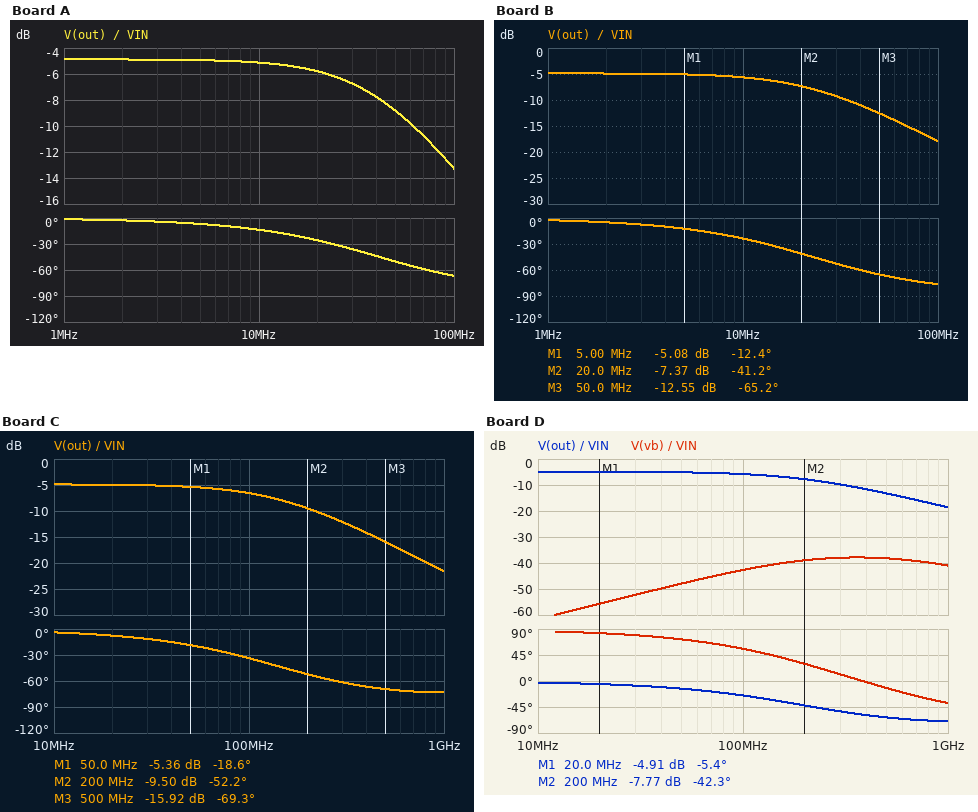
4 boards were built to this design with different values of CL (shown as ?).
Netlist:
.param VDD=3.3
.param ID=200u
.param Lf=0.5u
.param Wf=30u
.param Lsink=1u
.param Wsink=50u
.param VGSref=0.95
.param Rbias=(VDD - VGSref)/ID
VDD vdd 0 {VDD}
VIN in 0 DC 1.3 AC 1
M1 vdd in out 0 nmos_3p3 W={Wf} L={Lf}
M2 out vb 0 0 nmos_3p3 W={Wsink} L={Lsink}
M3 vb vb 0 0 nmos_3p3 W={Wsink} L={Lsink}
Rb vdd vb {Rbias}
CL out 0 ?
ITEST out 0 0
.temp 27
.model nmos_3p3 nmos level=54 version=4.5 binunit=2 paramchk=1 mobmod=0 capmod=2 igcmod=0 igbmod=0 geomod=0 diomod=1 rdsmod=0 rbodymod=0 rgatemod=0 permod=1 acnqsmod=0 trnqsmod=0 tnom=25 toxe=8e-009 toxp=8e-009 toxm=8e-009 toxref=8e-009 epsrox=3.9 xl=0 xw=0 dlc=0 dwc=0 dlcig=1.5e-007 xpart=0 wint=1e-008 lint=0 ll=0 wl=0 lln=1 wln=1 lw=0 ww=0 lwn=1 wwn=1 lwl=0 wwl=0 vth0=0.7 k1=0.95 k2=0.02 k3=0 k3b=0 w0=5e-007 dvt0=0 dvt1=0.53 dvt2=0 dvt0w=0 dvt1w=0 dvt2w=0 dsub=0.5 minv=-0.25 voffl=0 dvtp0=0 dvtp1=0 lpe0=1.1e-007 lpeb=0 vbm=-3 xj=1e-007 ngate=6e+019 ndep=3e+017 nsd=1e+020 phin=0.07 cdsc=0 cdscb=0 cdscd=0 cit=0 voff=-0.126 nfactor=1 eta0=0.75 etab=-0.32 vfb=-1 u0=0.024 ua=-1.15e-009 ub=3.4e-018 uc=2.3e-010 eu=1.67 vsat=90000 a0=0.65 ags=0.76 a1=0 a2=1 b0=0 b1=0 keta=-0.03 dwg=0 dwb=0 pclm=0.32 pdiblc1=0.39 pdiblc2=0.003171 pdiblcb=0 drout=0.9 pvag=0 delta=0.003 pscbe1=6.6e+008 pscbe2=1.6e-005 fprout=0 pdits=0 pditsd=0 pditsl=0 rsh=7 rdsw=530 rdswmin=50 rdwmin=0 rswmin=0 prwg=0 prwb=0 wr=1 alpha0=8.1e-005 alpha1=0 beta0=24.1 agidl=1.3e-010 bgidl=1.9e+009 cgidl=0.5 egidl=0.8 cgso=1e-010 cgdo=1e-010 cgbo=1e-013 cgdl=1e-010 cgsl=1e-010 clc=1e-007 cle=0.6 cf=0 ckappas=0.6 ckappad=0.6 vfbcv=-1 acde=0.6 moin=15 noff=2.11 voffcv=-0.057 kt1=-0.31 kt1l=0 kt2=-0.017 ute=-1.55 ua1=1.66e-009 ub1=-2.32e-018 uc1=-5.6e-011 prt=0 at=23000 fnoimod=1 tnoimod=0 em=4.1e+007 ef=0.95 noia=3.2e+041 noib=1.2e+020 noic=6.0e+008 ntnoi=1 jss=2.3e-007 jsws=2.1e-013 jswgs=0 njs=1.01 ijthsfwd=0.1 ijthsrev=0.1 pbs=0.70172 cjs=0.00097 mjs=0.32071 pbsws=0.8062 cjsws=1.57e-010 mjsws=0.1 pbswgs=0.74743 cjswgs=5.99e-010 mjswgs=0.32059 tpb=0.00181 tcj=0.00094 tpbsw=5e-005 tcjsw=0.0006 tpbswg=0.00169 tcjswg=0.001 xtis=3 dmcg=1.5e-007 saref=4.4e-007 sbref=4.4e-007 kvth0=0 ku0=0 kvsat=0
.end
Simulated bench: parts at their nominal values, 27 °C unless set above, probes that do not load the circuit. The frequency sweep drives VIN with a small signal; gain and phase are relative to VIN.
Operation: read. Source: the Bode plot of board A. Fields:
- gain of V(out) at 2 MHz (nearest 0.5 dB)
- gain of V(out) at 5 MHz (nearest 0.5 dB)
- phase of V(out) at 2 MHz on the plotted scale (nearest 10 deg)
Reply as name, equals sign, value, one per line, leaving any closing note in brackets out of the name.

gain of V(out) at 2 MHz = -5.0 dB
gain of V(out) at 5 MHz = -5.0 dB
phase of V(out) at 2 MHz on the plotted scale = 0 deg
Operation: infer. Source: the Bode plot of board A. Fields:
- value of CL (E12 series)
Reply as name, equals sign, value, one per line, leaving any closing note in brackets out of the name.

value of CL = 8.2 pF
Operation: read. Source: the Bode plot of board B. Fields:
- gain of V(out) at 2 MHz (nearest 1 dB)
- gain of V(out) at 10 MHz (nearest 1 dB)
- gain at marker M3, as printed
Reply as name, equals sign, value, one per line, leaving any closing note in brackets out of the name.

gain of V(out) at 2 MHz = -5 dB
gain of V(out) at 10 MHz = -6 dB
gain at marker M3, as printed = -12.55 dB
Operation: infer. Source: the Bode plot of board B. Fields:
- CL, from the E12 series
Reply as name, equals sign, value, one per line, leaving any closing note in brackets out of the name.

CL, from the E12 series = 15 pF
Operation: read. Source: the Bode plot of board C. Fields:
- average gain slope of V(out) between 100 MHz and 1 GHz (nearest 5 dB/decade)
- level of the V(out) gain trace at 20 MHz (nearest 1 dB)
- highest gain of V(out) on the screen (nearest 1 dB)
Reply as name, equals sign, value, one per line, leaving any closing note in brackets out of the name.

average gain slope of V(out) between 100 MHz and 1 GHz = -15 dB/decade
level of the V(out) gain trace at 20 MHz = -5 dB
highest gain of V(out) on the screen = -5 dB
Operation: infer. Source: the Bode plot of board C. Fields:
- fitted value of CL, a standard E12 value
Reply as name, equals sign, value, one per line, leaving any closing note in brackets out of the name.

fitted value of CL, a standard E12 value = 2.2 pF
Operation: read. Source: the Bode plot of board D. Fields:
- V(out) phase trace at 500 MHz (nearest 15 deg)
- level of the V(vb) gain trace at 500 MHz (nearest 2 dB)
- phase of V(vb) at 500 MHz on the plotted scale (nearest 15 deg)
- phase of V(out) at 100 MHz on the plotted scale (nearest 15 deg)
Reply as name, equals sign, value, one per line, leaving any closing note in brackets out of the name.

V(out) phase trace at 500 MHz = -60 deg
level of the V(vb) gain trace at 500 MHz = -38 dB
phase of V(vb) at 500 MHz on the plotted scale = -15 deg
phase of V(out) at 100 MHz on the plotted scale = -30 deg
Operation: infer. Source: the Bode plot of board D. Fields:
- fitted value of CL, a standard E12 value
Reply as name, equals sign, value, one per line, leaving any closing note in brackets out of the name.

fitted value of CL, a standard E12 value = 1.5 pF
